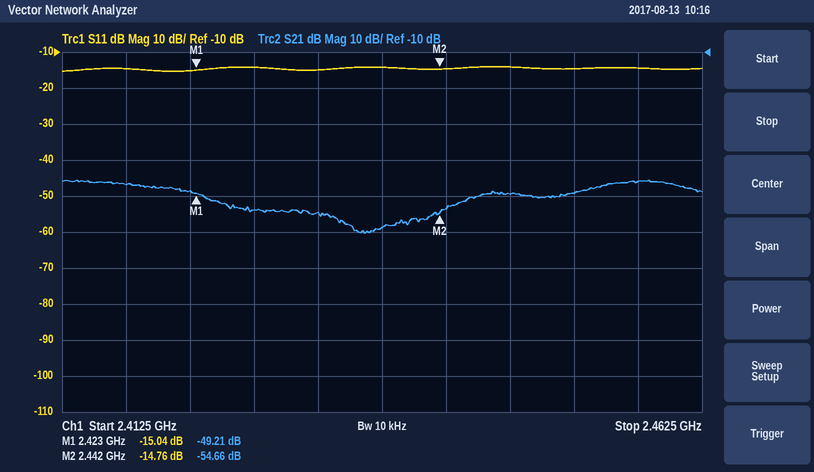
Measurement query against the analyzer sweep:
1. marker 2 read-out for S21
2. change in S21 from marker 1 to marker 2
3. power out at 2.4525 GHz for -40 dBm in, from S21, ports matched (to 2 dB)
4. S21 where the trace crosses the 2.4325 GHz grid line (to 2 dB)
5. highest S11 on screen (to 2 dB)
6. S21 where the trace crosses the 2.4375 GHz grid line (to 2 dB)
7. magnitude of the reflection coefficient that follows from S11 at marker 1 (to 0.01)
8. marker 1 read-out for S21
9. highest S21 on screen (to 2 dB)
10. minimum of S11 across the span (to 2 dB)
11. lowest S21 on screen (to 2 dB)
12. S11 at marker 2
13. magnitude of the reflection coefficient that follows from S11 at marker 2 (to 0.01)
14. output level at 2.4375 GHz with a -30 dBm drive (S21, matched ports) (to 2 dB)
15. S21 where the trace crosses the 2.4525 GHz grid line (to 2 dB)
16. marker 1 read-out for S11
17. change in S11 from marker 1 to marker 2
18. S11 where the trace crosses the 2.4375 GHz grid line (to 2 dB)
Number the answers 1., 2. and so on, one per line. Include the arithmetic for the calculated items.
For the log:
1. -54.66 dB
2. -54.66 − (-49.21) = -5.45 dB
3. -40 dBm + (-50 dB) = -90 dBm
4. -54 dB
5. -14 dB
6. -58 dB
7. 10^(-15.04/20) ≈ 0.18
8. -49.21 dB
9. -46 dB
10. -16 dB
11. -60 dB
12. -14.76 dB
13. 10^(-14.76/20) ≈ 0.18
14. -30 dBm + (-58 dB) = -88 dBm
15. -50 dB
16. -15.04 dB
17. -14.76 − (-15.04) = 0.28 dB
18. -14 dB
